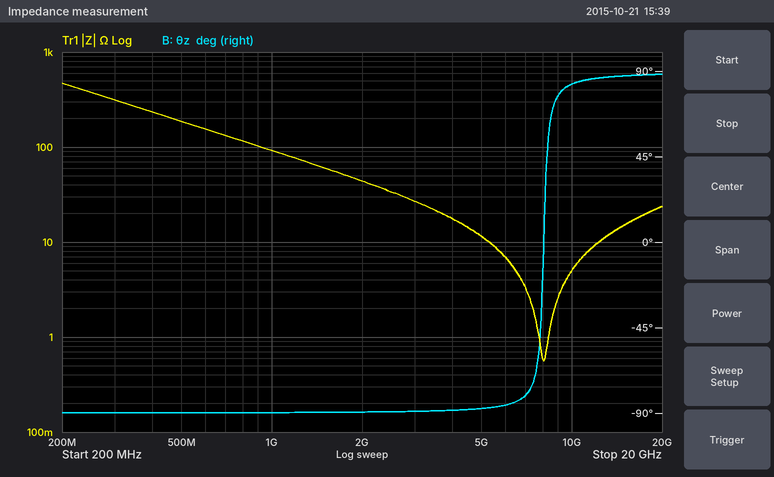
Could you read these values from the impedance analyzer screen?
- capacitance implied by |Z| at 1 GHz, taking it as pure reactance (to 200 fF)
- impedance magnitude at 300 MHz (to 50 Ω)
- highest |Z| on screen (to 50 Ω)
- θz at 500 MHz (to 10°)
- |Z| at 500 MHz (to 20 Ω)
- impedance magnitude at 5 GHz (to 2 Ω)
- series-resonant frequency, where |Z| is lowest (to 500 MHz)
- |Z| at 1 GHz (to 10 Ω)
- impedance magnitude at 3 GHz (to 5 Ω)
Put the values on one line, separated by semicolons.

1.8 pF; 300 Ω; 450 Ω; -90°; 180 Ω; 12 Ω; 8.0 GHz; 90 Ω; 25 Ω
